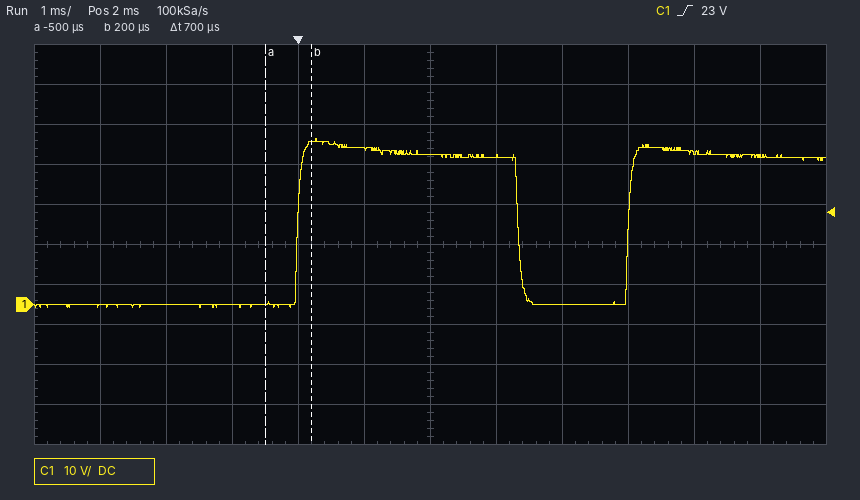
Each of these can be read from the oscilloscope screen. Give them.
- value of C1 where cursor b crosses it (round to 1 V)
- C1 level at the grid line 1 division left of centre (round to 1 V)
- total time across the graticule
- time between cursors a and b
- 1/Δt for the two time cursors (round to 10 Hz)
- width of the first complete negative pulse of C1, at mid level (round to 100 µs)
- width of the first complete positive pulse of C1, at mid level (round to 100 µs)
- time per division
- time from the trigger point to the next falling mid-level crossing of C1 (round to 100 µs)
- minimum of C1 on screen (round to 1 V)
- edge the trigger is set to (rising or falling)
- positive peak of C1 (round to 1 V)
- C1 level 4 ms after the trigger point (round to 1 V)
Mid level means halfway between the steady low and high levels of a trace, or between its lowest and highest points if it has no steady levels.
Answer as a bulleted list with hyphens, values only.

- 40 V
- 39 V
- 12 ms
- 700 µs
- 1.43 kHz
- 1.7 ms
- 3.3 ms
- 1 ms
- 3.3 ms
- -1 V
- rising
- 42 V
- 0 V
